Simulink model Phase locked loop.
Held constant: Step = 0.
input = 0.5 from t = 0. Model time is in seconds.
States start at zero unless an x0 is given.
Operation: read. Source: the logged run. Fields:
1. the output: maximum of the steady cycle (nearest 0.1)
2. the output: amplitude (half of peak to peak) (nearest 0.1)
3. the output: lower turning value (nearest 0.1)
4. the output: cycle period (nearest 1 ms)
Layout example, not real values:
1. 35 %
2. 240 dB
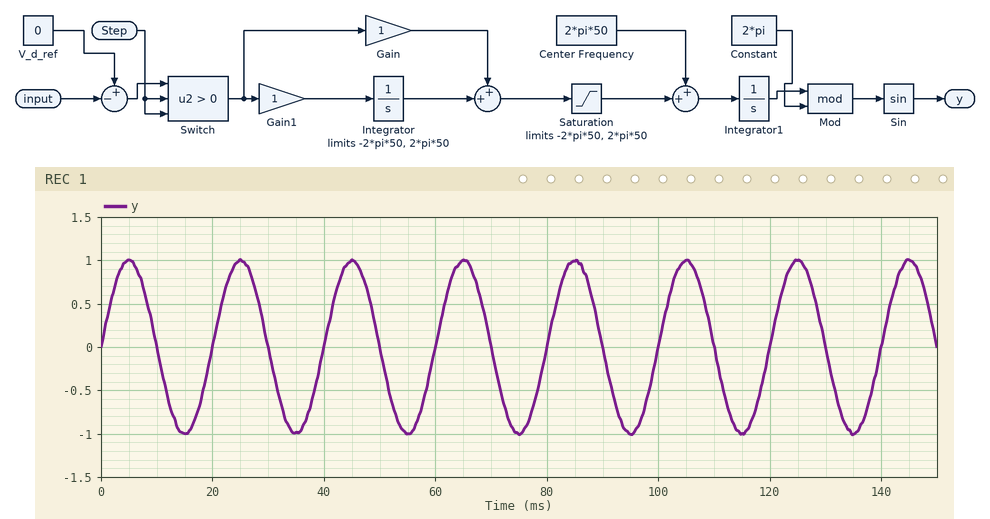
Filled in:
1. 1.0
2. 1.0
3. -1.0
4. 20 ms
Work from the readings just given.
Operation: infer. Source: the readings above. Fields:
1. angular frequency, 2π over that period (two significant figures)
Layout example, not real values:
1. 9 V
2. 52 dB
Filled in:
1. 0.31 rad/ms
